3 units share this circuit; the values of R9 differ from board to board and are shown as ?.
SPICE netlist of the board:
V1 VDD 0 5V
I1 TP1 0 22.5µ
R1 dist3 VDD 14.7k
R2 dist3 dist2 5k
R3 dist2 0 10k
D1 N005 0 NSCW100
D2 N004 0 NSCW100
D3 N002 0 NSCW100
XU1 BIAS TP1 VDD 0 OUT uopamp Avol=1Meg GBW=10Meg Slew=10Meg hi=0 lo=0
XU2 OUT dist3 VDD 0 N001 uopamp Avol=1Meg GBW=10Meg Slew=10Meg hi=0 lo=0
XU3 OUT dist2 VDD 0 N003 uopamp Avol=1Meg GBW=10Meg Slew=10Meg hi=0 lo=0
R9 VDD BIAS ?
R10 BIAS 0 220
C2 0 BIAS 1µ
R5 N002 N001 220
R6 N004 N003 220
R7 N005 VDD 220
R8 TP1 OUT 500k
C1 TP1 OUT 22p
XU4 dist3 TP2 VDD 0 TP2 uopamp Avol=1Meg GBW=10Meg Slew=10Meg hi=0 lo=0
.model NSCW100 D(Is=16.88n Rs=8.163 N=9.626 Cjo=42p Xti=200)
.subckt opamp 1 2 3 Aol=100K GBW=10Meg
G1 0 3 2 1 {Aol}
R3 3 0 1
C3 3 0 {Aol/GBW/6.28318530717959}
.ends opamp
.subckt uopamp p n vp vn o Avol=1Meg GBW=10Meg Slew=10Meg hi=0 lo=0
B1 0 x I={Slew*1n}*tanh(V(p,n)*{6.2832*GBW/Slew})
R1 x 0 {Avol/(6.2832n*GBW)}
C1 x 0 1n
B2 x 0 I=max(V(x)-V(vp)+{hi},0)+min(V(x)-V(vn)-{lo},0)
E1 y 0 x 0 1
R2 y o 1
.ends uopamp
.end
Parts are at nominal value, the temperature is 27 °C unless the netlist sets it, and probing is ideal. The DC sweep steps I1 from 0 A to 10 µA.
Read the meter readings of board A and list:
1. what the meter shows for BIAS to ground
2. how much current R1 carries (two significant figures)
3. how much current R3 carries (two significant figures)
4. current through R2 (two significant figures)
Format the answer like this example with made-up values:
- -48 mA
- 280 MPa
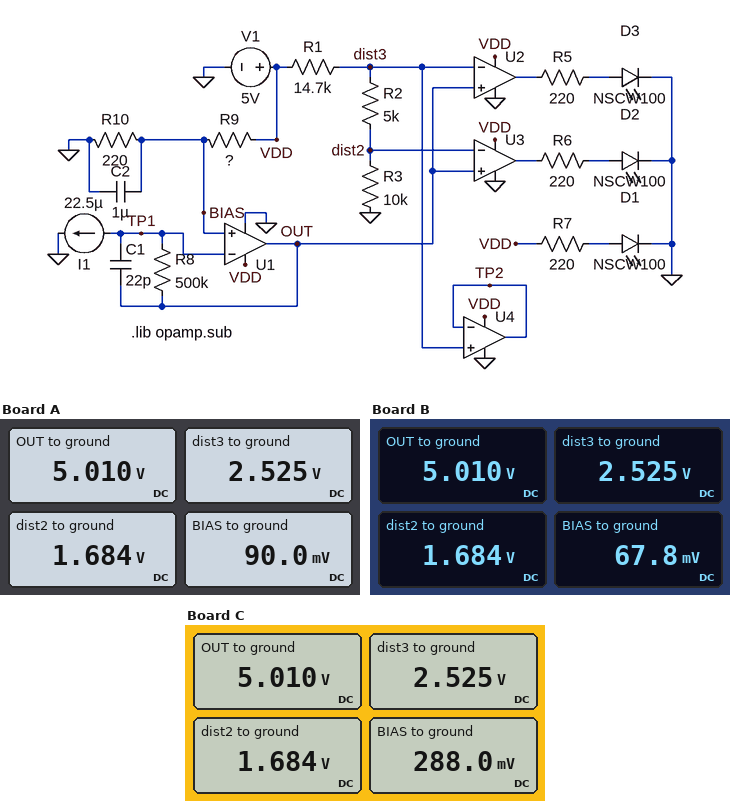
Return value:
- 90.0 mV
- 170 µA
- 170 µA
- 170 µA
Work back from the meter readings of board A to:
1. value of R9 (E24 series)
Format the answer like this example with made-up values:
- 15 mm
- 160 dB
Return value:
- 12 kΩ
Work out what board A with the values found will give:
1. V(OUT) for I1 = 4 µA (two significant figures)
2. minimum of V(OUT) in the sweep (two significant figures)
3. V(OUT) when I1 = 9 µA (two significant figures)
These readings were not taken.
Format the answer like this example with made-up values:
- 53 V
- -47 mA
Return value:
- 2.1 V
- 90 mV
- 4.6 V
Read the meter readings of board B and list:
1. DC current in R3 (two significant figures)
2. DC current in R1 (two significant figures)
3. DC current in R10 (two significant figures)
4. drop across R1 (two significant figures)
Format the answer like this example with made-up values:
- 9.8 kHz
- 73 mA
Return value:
- 170 µA
- 170 µA
- 310 µA
- 2.5 V
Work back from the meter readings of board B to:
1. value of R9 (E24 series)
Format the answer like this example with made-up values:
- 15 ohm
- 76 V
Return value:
- 16 kΩ
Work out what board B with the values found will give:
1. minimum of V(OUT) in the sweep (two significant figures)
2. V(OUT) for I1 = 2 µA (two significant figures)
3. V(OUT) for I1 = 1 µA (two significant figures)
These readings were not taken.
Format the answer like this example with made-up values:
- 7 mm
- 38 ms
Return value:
- 68 mV
- 1.1 V
- 570 mV
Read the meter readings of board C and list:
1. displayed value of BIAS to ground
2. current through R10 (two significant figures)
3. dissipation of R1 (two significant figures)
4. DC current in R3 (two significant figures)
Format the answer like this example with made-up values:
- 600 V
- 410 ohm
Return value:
- 288.0 mV
- 1.3 mA
- 420 µW
- 170 µA
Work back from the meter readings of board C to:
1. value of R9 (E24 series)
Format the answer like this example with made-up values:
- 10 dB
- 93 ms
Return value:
- 3.6 kΩ
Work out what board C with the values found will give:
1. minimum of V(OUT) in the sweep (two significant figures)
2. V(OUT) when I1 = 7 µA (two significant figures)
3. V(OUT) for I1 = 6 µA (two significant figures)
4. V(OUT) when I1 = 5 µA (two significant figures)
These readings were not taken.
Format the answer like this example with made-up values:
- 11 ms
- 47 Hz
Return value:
- 290 mV
- 3.8 V
- 3.3 V
- 2.8 V
